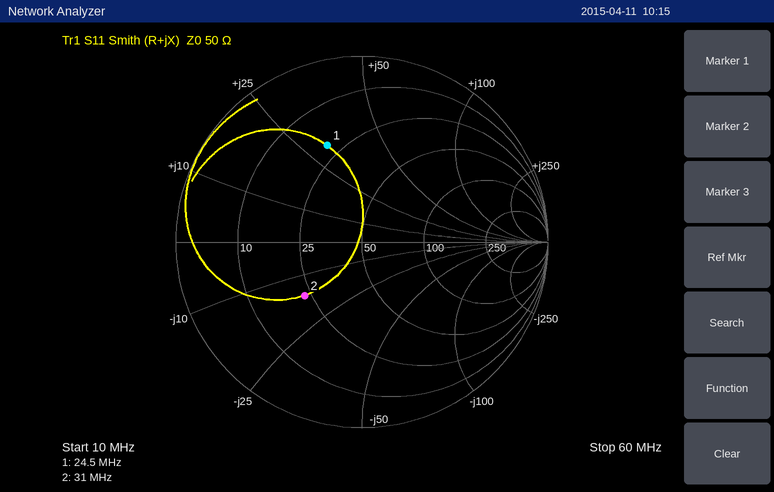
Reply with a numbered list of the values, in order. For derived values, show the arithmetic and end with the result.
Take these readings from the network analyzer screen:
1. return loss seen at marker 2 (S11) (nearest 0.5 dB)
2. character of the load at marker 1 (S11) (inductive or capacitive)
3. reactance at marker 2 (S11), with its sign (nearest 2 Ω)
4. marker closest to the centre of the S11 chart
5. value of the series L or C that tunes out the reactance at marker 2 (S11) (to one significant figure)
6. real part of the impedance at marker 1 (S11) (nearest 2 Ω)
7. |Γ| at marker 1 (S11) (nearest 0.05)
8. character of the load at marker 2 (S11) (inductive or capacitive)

1. 7.5 dB
2. inductive
3. -16 Ω
4. marker 2
5. L = 16 Ω/(2π × 31 MHz) ≈ 82.1 nH, so 80 nH to one significant figure
6. 20 Ω
7. 0.55
8. capacitive
